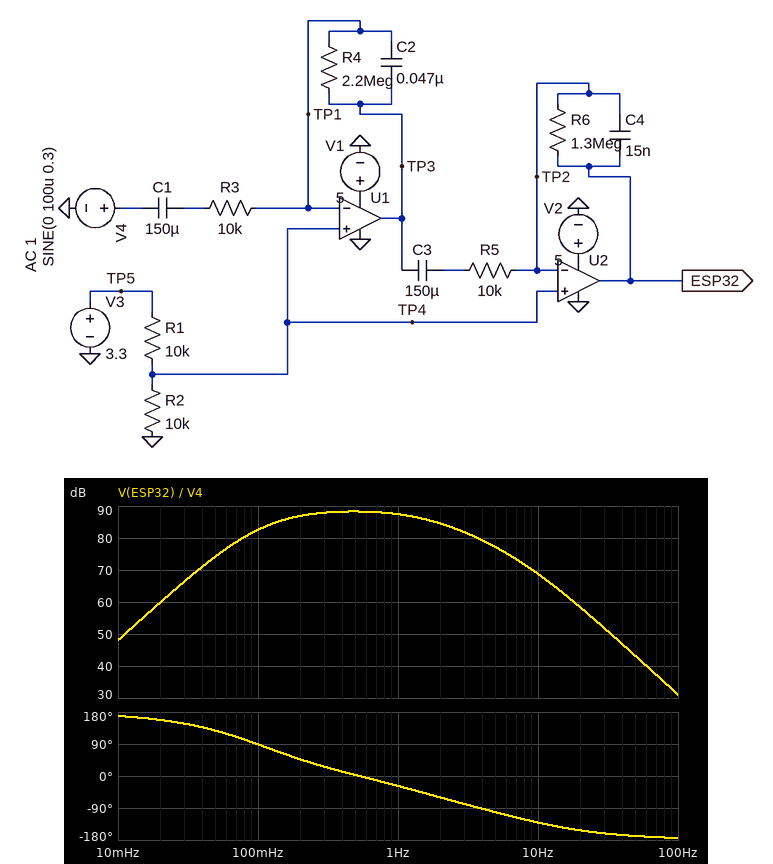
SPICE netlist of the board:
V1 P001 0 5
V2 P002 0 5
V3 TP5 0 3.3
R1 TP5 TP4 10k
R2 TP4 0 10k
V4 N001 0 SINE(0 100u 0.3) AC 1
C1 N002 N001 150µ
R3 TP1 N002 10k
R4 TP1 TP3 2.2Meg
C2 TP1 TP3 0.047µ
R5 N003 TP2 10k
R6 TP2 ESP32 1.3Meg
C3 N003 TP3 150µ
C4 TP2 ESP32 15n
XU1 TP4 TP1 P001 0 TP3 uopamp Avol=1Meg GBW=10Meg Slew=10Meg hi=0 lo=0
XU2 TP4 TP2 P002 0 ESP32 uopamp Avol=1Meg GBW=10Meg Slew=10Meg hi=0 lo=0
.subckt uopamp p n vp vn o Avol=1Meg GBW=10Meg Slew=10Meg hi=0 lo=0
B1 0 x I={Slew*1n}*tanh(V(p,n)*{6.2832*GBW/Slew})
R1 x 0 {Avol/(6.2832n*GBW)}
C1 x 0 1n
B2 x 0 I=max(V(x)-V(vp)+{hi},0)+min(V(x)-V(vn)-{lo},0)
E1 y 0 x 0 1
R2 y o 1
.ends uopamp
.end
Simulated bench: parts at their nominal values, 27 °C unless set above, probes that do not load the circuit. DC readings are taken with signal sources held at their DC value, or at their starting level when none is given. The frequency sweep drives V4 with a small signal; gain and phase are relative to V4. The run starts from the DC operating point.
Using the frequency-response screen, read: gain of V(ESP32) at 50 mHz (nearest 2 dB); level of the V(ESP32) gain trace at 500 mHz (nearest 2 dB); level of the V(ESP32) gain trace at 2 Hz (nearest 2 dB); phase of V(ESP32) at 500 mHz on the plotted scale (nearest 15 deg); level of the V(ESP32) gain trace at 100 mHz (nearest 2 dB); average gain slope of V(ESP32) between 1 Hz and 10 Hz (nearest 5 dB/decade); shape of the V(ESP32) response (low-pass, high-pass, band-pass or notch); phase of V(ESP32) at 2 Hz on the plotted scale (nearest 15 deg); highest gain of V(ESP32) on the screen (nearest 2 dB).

74 dB
88 dB
84 dB
0 deg
82 dB
-20 dB/decade
band-pass
-60 deg
88 dB
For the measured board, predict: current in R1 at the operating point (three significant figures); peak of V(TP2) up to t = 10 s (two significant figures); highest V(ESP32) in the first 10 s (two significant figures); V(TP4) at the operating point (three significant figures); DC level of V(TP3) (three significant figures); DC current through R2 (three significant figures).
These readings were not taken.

165 µA
1.7 V
4.0 V
1.65 V
1.65 V
165 µA
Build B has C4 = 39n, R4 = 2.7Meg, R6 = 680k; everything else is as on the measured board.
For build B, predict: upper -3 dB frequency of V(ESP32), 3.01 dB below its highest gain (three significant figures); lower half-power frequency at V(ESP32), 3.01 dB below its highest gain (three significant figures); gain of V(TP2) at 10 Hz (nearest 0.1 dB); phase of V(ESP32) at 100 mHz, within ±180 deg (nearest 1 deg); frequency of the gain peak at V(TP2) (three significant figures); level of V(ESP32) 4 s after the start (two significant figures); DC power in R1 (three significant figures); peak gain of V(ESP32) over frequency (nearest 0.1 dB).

1.46 Hz
139 mHz
-55.6 dB
88 deg
437 mHz
3.3 V
272 µW
84.3 dB
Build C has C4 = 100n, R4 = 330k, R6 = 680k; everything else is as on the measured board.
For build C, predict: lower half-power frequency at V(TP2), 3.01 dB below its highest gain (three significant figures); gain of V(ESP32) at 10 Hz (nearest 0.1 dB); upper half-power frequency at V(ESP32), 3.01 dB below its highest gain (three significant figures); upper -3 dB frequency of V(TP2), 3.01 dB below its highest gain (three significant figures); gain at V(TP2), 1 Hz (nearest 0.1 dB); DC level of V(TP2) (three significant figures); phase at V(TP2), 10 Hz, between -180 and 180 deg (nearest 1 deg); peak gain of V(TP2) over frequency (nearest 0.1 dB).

150 mHz
51.3 dB
2.50 Hz
2.63 Hz
-53.8 dB
1.65 V
105 deg
-53.5 dB
